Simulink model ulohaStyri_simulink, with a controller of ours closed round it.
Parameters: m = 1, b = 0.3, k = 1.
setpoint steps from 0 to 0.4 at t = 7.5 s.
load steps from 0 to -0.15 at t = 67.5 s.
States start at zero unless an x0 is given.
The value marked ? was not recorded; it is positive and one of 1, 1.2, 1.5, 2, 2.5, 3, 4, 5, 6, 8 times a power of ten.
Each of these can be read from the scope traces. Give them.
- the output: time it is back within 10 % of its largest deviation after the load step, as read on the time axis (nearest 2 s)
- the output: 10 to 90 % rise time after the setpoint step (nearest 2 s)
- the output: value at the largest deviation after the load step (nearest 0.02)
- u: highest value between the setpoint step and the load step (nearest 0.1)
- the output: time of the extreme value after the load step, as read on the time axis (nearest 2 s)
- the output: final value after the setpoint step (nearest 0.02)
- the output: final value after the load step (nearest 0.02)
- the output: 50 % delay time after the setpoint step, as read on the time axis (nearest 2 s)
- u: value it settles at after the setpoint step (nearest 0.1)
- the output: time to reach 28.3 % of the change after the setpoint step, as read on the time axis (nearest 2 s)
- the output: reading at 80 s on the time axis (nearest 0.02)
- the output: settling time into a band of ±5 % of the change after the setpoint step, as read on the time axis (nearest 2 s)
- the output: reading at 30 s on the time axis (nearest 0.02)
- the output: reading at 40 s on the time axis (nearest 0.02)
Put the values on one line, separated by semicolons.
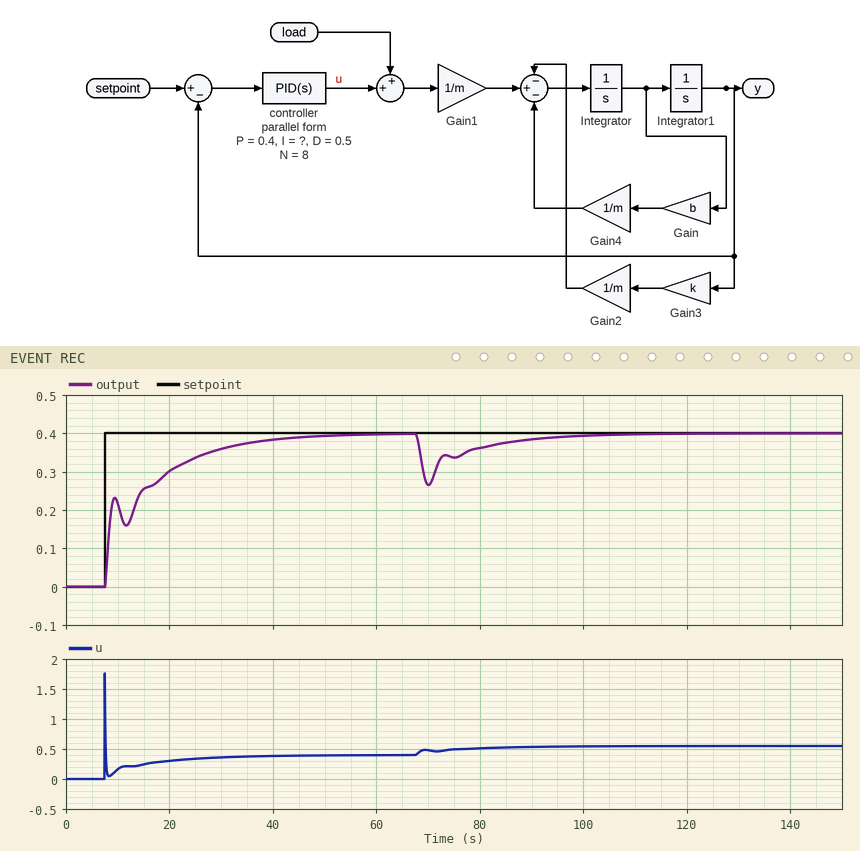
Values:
92 s; 22 s; 0.26; 1.8; 70 s; 0.40; 0.40; 8 s; 0.4; 8 s; 0.36; 38 s; 0.36; 0.38
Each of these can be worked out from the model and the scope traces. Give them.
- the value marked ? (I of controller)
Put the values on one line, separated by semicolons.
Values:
0.12
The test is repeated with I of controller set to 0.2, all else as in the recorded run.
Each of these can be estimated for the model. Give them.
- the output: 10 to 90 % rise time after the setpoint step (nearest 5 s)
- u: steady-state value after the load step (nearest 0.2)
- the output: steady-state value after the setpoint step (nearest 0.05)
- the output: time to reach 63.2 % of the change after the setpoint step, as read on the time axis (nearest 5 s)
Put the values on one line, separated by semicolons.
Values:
15 s; 0.6; 0.40; 15 s
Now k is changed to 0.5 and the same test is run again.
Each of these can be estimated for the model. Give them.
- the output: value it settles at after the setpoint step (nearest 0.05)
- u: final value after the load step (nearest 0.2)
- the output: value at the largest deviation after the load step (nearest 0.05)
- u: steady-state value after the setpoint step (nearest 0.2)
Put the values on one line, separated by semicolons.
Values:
0.40; 0.4; 0.20; 0.2
